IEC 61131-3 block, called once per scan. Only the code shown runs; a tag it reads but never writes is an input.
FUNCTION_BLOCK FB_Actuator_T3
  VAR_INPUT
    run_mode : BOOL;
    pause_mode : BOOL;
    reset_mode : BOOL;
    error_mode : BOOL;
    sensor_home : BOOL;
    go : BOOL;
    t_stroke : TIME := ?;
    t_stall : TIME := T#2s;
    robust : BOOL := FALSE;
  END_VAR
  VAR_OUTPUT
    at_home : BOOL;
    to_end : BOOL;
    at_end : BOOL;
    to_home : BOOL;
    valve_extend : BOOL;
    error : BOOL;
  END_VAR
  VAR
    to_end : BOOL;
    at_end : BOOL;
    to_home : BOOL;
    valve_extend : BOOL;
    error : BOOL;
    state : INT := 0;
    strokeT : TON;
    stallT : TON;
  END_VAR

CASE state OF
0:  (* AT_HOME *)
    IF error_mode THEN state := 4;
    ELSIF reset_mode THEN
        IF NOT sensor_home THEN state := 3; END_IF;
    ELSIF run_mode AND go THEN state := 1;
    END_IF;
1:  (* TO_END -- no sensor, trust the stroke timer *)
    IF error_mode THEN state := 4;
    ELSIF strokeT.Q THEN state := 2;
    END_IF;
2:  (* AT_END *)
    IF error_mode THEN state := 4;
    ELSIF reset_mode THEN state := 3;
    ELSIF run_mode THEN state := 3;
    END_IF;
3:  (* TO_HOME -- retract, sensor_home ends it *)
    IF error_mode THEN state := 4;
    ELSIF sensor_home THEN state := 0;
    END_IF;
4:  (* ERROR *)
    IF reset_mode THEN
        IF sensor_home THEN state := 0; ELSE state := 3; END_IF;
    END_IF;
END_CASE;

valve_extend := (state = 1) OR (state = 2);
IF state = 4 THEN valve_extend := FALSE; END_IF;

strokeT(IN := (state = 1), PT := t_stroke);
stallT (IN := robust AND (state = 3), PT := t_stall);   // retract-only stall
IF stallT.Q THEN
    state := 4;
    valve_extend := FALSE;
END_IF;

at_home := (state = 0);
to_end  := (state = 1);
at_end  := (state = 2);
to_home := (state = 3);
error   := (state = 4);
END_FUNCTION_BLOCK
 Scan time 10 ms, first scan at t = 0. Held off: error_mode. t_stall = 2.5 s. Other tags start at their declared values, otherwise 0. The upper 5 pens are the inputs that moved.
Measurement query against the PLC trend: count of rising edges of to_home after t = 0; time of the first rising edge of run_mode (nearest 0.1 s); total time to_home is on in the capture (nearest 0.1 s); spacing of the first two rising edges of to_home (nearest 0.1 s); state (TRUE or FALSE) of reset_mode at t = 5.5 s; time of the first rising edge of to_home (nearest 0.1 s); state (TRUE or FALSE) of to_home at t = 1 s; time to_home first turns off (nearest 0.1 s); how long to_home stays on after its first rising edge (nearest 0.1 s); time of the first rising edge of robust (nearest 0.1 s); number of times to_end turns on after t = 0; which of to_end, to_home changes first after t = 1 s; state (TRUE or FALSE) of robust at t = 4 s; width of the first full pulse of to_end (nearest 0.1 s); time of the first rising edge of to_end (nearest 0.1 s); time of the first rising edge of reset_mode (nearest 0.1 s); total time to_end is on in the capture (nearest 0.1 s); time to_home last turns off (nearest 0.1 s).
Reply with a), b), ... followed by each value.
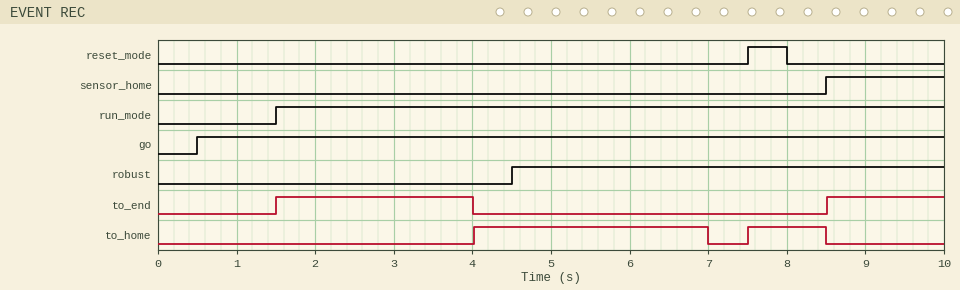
a) 2
b) 1.5 s
c) 4.0 s
d) 3.5 s
e) FALSE
f) 4.0 s
g) FALSE
h) 7.0 s
i) 3.0 s
j) 4.5 s
k) 2
l) to_end
m) FALSE
n) 2.5 s
o) 1.5 s
p) 7.5 s
q) 4.0 s
r) 8.5 s
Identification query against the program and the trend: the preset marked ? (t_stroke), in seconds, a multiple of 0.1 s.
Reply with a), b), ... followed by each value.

a) 2.5 s
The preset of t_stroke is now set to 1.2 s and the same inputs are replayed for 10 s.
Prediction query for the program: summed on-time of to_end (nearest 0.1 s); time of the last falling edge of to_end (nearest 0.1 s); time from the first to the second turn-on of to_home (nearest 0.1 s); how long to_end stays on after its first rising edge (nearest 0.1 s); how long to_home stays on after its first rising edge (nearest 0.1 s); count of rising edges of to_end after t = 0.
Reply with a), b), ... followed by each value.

a) 2.7 s
b) 9.7 s
c) 4.8 s
d) 1.2 s
e) 4.3 s
f) 3
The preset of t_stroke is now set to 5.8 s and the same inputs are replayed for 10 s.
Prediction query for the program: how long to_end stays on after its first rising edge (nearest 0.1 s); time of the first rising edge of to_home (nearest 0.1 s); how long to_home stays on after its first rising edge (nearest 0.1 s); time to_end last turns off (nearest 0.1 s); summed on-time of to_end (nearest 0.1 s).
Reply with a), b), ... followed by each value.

a) 5.8 s
b) 7.3 s
c) 1.2 s
d) 7.3 s
e) 7.3 s
